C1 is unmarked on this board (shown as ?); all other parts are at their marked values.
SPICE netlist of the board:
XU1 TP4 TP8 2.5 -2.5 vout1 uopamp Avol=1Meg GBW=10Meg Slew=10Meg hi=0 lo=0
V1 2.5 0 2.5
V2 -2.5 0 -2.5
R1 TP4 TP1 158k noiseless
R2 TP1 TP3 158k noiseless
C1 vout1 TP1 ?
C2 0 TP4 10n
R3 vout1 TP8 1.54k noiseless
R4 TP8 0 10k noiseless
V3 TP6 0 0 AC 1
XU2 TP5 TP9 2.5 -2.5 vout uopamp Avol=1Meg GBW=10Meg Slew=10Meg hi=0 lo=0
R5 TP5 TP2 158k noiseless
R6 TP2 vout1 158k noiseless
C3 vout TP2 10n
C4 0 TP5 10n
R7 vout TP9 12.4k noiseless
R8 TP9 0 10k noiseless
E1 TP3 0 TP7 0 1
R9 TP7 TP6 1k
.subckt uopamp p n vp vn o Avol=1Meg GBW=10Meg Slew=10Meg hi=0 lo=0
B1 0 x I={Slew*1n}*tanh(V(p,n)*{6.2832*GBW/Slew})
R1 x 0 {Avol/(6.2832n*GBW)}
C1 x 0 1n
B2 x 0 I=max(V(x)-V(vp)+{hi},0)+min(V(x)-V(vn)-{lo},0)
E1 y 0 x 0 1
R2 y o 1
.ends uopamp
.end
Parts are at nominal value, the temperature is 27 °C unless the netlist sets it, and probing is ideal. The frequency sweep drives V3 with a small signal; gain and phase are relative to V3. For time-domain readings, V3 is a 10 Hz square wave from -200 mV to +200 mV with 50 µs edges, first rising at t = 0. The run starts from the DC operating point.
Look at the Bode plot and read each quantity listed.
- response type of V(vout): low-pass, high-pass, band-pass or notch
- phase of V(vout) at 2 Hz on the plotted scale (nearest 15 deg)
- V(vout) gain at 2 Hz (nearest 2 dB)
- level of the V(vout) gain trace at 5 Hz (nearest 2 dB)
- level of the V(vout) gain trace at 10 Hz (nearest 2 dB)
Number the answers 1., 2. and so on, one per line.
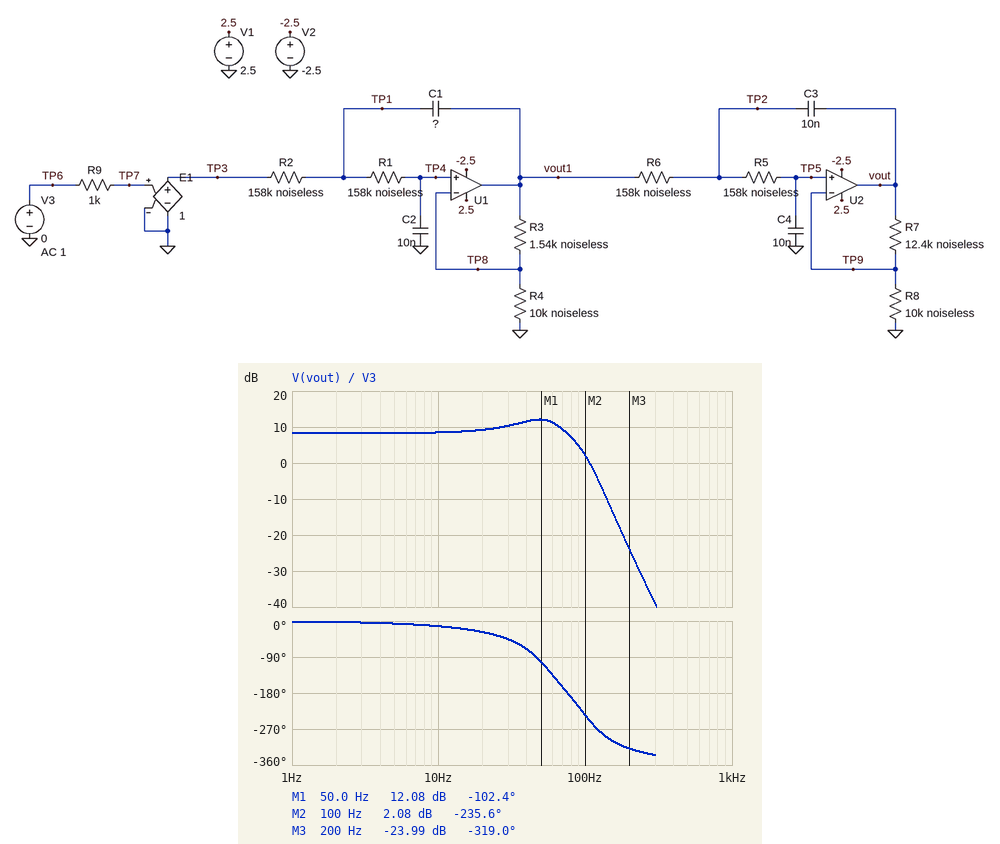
1. low-pass
2. 0 deg
3. 8 dB
4. 8 dB
5. 8 dB
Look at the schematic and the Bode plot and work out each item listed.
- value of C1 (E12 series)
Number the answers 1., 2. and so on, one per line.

1. 33 nF
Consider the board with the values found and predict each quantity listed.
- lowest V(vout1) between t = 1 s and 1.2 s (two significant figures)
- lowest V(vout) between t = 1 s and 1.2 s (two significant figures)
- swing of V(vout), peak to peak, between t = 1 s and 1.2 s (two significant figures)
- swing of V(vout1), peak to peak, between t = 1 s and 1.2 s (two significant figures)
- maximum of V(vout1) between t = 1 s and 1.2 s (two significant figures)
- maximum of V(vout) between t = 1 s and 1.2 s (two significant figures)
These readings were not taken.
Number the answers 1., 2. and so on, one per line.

1. -340 mV
2. -890 mV
3. 1.8 V
4. 690 mV
5. 340 mV
6. 890 mV
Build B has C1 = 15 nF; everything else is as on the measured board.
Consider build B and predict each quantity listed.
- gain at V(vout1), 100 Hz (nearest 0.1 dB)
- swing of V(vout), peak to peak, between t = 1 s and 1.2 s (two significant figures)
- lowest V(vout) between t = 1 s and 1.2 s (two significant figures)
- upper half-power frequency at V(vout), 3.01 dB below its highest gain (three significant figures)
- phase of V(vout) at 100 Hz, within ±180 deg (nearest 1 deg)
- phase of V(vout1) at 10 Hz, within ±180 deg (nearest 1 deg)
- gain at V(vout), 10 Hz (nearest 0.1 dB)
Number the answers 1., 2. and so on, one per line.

1. -4.0 dB
2. 1.4 V
3. -700 mV
4. 96.9 Hz
5. 166 deg
6. -10 deg
7. 8.3 dB
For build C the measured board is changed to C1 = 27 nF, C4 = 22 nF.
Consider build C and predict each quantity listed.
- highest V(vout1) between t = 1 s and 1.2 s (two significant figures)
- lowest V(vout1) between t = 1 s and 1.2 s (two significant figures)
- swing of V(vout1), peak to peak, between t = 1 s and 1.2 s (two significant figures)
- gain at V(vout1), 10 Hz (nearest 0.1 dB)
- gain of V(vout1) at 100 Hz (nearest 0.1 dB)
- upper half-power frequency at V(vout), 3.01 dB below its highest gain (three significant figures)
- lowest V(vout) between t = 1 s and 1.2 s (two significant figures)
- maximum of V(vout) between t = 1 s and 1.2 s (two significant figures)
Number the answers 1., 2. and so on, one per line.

1. 310 mV
2. -310 mV
3. 630 mV
4. 1.4 dB
5. -5.9 dB
6. 50.6 Hz
7. -550 mV
8. 550 mV
